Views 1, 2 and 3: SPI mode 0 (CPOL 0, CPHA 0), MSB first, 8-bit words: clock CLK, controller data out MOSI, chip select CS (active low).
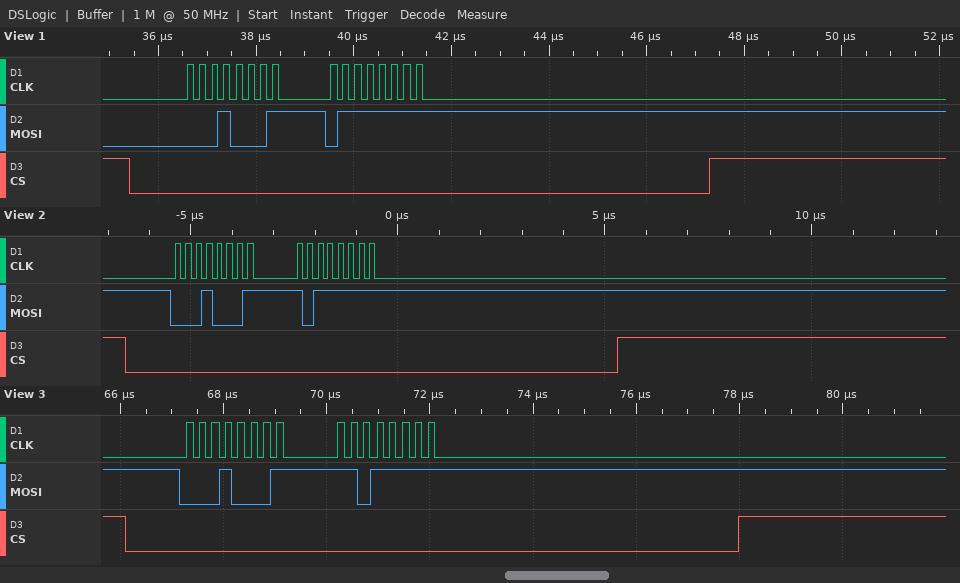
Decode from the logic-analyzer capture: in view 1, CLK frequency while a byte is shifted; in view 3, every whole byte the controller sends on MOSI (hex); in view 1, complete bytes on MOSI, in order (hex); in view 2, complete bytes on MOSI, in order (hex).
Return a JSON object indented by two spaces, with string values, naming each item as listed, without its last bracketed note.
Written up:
{
  "in view 1, CLK frequency while a byte is shifted": "4 MHz",
  "in view 3, every whole byte the controller sends on MOSI": "11 DF",
  "in view 1, complete bytes on MOSI, in order": "11 7F",
  "in view 2, complete bytes on MOSI, in order": "11 BF"
}
